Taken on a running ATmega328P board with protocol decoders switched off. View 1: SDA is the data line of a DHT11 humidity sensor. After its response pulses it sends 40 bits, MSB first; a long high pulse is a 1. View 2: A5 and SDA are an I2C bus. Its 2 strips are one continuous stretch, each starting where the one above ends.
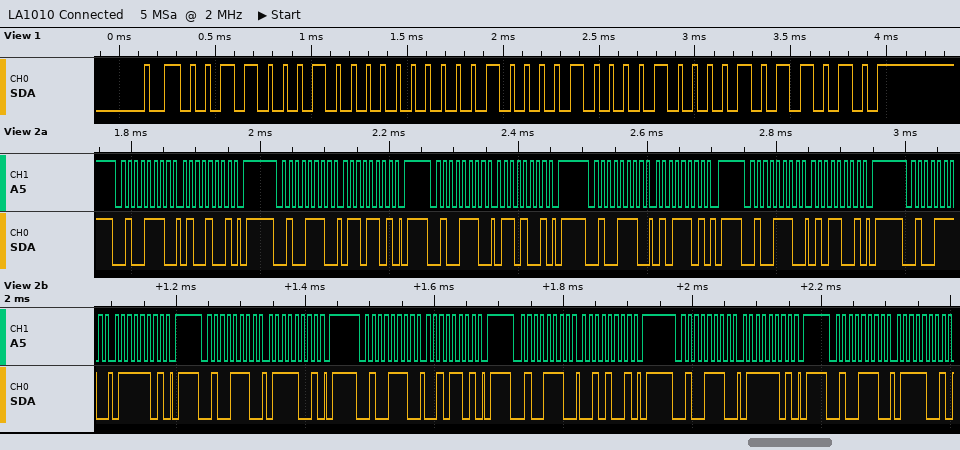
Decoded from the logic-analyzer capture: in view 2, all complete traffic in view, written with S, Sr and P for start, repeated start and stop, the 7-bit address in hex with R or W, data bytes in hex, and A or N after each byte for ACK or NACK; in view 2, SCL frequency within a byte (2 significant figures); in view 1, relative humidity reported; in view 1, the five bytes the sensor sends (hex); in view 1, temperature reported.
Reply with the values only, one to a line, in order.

S 27W A 49 A P S 27W A 6D A P S 27W A 69 A P S 27W A 5D A P S 27W A 59 A P S 27W A 7D A P S 27W A 79 A P S 27W A 2D A P S 27W A 29 A P S 27W A 7D A P S 27W A 79 A
100 kHz
49 %
31 00 21 08 5A
33.8 °C
